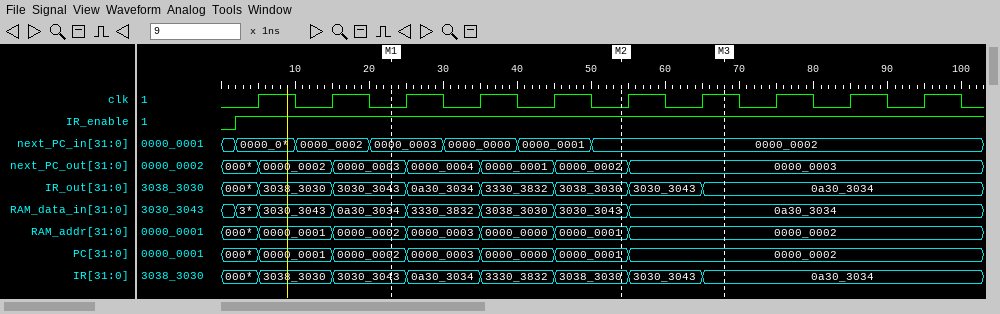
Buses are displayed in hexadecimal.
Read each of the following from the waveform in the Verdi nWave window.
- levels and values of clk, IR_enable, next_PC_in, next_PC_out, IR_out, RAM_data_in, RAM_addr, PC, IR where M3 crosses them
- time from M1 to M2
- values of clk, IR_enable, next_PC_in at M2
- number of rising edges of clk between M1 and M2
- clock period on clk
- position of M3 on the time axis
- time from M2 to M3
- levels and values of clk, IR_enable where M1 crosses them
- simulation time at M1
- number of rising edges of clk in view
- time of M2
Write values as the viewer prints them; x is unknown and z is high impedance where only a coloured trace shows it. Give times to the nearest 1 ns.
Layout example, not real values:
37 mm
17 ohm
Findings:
clk=1, IR_enable=1, next_PC_in=0000_0002, next_PC_out=0000_0003, IR_out=0a30_3034, RAM_data_in=0a30_3034, RAM_addr=0000_0002, PC=0000_0002, IR=0a30_3034
31 ns
clk=0, IR_enable=1, next_PC_in=0000_0002
3
10 ns
68 ns
14 ns
clk=0, IR_enable=1
23 ns
10
54 ns
